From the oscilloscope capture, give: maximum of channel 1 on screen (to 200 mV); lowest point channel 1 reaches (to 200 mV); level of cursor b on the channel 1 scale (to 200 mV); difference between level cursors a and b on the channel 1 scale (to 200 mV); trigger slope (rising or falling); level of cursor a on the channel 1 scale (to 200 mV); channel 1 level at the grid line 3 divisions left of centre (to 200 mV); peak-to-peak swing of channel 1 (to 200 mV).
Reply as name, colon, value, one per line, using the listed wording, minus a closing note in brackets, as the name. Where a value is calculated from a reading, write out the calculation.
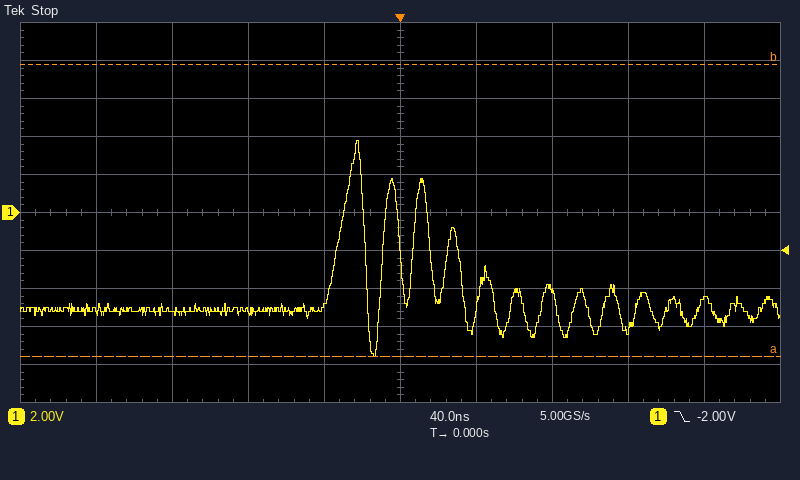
maximum of channel 1 on screen: 3.8 V
lowest point channel 1 reaches: -7.6 V
level of cursor b on the channel 1 scale: 7.8 V
difference between level cursors a and b on the channel 1 scale: 15.4 V
trigger slope: falling
level of cursor a on the channel 1 scale: -7.6 V
channel 1 level at the grid line 3 divisions left of centre: -5.2 V
peak-to-peak swing of channel 1: 3.8 V − (-7.6 V) = 11.4 V
